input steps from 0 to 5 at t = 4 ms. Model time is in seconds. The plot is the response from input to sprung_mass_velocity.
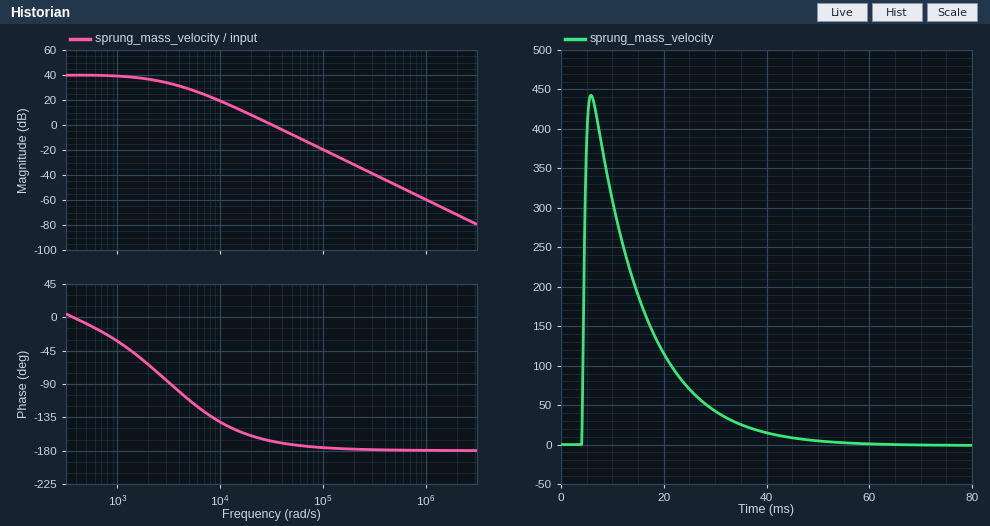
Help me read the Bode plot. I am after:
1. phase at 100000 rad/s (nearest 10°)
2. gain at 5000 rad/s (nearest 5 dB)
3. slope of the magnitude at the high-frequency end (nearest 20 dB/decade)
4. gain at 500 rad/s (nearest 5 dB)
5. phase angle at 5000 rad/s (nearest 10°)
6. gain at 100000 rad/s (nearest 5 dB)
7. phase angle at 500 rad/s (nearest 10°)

-180°
30 dB
-40 dB/decade
40 dB
-110°
-20 dB
-10°
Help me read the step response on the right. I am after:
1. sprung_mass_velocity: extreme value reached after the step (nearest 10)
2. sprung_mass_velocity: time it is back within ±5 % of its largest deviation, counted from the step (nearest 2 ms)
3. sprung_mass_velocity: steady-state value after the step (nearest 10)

440
32 ms
0
